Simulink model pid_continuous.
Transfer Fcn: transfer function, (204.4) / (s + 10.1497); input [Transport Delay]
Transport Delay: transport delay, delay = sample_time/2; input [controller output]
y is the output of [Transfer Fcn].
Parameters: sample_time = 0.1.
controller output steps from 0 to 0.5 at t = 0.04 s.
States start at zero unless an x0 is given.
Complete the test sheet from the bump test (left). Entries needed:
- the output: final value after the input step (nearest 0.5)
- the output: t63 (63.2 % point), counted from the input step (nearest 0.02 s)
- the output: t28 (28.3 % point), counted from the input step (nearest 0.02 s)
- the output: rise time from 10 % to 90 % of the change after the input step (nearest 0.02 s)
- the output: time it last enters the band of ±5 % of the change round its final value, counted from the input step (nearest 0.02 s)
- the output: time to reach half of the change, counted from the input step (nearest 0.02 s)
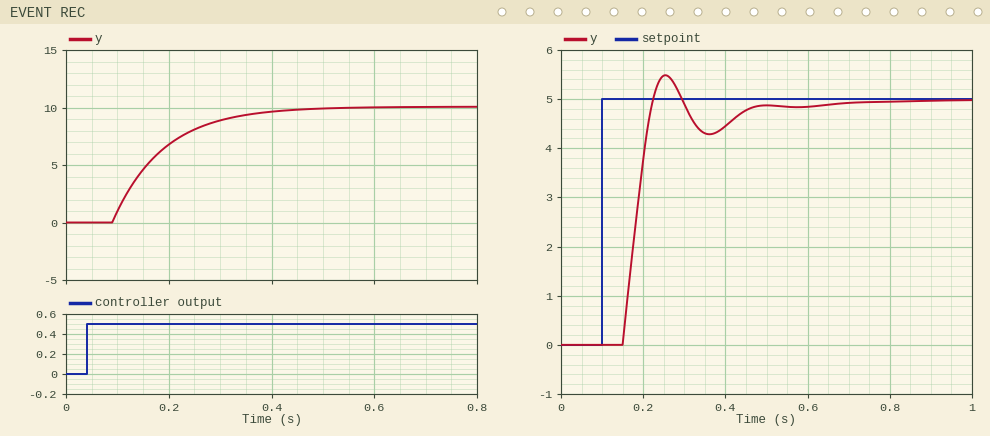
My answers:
10.0
0.14 s
0.08 s
0.22 s
0.34 s
0.12 s
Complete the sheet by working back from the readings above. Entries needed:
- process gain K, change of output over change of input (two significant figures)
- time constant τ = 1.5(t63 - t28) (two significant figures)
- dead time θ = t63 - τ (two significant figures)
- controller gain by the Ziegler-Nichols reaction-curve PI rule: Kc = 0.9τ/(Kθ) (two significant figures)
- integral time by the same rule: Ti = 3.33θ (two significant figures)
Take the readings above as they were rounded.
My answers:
20
0.090 s
0.050 s
0.081
0.17 s
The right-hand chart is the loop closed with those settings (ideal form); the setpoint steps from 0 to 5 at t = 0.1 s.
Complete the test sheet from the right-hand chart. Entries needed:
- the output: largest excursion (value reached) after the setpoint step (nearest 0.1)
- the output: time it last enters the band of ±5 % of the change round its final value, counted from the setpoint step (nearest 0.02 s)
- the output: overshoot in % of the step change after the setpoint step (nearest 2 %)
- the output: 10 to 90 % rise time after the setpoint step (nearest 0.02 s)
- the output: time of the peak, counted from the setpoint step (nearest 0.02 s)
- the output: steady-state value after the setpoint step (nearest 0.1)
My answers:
5.5
0.34 s
10 %
0.06 s
0.16 s
5.0
